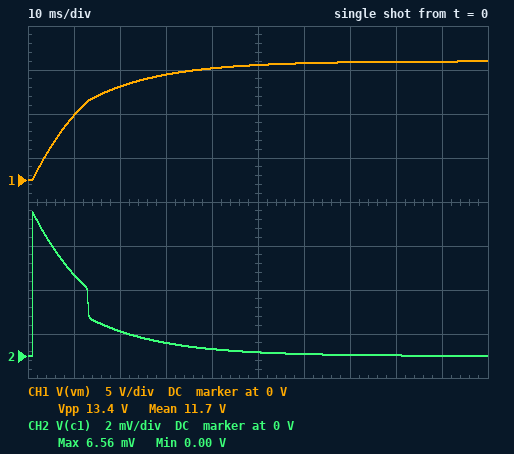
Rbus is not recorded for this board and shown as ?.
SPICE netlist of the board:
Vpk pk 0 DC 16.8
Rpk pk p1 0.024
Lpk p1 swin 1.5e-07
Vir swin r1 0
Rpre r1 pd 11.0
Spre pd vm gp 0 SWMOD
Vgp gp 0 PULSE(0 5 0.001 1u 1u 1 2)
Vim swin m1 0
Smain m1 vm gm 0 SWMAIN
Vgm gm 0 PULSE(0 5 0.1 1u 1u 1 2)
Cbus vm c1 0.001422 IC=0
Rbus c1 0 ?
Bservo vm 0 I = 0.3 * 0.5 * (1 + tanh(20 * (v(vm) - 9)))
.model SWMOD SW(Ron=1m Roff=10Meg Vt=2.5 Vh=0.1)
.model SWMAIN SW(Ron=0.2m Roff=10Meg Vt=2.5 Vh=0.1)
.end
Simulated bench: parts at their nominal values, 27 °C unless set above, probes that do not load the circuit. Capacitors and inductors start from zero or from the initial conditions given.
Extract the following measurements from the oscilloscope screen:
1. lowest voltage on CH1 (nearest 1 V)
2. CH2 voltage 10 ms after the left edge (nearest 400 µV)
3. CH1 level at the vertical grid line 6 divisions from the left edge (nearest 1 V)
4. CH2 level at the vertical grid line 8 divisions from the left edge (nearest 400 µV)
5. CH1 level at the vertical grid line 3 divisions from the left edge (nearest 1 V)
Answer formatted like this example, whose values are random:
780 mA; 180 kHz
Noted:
0 V; 3.6 mV; 13 V; 0 V; 12 V
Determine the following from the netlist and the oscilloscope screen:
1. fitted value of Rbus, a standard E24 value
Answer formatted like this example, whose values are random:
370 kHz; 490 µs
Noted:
4.3 mΩ
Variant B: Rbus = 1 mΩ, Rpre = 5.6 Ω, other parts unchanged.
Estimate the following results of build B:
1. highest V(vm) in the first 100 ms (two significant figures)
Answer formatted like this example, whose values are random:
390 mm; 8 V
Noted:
15 V
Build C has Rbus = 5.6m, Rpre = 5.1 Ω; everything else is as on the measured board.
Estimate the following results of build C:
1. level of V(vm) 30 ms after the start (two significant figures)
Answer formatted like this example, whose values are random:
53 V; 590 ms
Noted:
15 V
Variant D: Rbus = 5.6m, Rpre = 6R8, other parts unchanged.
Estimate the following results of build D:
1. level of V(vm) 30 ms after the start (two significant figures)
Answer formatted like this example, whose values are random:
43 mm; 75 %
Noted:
14 V
